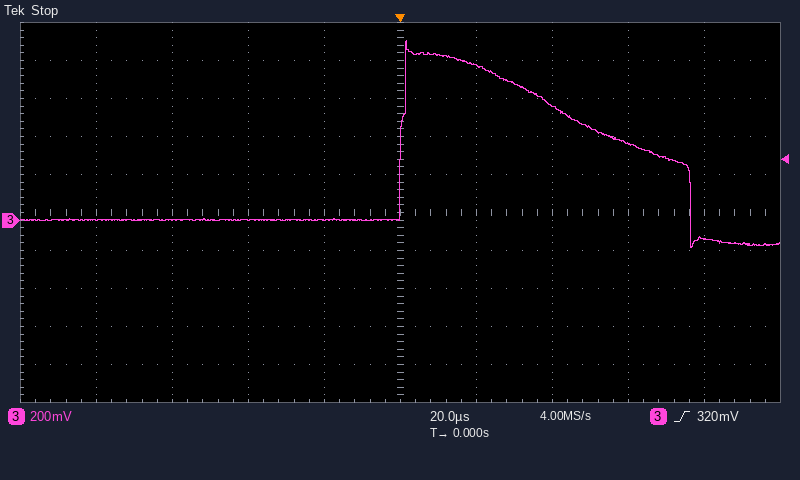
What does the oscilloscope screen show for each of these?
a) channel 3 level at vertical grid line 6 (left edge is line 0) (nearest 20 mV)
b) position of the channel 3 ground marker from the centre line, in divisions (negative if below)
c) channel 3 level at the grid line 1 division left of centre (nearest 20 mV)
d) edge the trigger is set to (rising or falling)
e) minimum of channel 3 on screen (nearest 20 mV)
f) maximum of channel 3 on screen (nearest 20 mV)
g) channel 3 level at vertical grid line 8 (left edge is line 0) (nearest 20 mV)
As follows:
820 mV
-0.2 div
0 mV
rising
-140 mV
940 mV
400 mV
